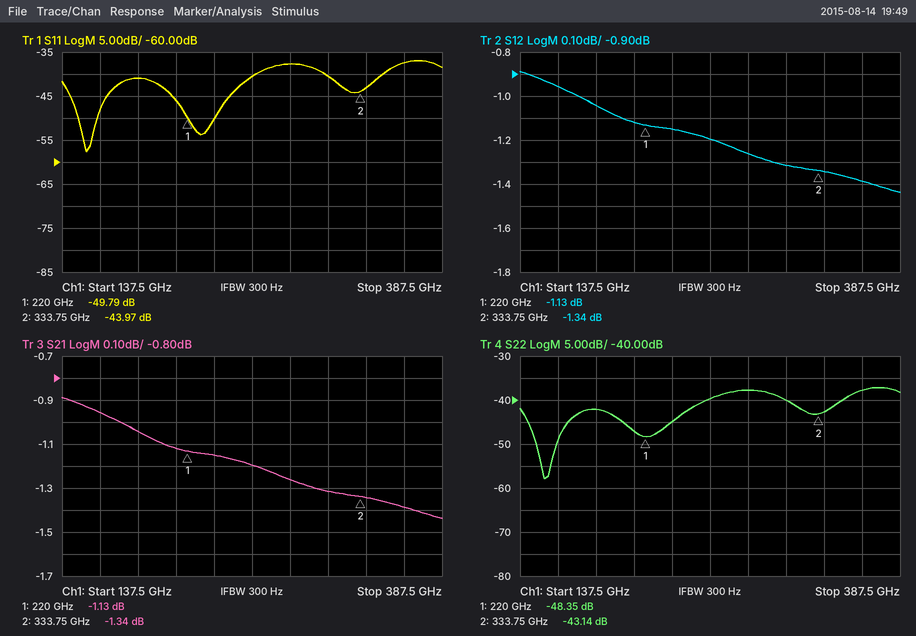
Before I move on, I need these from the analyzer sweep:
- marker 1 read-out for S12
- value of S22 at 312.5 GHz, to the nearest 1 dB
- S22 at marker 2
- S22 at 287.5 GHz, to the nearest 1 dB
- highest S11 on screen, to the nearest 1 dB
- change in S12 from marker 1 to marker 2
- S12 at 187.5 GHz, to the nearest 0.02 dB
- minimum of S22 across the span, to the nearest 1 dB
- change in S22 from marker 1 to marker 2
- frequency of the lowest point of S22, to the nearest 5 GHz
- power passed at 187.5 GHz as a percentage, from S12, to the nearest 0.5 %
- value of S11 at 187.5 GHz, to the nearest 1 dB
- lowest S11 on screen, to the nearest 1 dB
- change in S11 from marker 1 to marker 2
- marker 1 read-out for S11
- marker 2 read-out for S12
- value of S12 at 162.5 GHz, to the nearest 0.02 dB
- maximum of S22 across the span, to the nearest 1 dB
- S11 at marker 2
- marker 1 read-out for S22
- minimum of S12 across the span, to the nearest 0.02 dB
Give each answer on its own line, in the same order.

-1.13 dB
-40 dB
-43.14 dB
-38 dB
-37 dB
-0.21 dB
-1.04 dB
-58 dB
5.21 dB
155 GHz
78.5 %
-41 dB
-58 dB
5.82 dB
-49.79 dB
-1.34 dB
-0.96 dB
-37 dB
-43.97 dB
-48.35 dB
-1.44 dB
